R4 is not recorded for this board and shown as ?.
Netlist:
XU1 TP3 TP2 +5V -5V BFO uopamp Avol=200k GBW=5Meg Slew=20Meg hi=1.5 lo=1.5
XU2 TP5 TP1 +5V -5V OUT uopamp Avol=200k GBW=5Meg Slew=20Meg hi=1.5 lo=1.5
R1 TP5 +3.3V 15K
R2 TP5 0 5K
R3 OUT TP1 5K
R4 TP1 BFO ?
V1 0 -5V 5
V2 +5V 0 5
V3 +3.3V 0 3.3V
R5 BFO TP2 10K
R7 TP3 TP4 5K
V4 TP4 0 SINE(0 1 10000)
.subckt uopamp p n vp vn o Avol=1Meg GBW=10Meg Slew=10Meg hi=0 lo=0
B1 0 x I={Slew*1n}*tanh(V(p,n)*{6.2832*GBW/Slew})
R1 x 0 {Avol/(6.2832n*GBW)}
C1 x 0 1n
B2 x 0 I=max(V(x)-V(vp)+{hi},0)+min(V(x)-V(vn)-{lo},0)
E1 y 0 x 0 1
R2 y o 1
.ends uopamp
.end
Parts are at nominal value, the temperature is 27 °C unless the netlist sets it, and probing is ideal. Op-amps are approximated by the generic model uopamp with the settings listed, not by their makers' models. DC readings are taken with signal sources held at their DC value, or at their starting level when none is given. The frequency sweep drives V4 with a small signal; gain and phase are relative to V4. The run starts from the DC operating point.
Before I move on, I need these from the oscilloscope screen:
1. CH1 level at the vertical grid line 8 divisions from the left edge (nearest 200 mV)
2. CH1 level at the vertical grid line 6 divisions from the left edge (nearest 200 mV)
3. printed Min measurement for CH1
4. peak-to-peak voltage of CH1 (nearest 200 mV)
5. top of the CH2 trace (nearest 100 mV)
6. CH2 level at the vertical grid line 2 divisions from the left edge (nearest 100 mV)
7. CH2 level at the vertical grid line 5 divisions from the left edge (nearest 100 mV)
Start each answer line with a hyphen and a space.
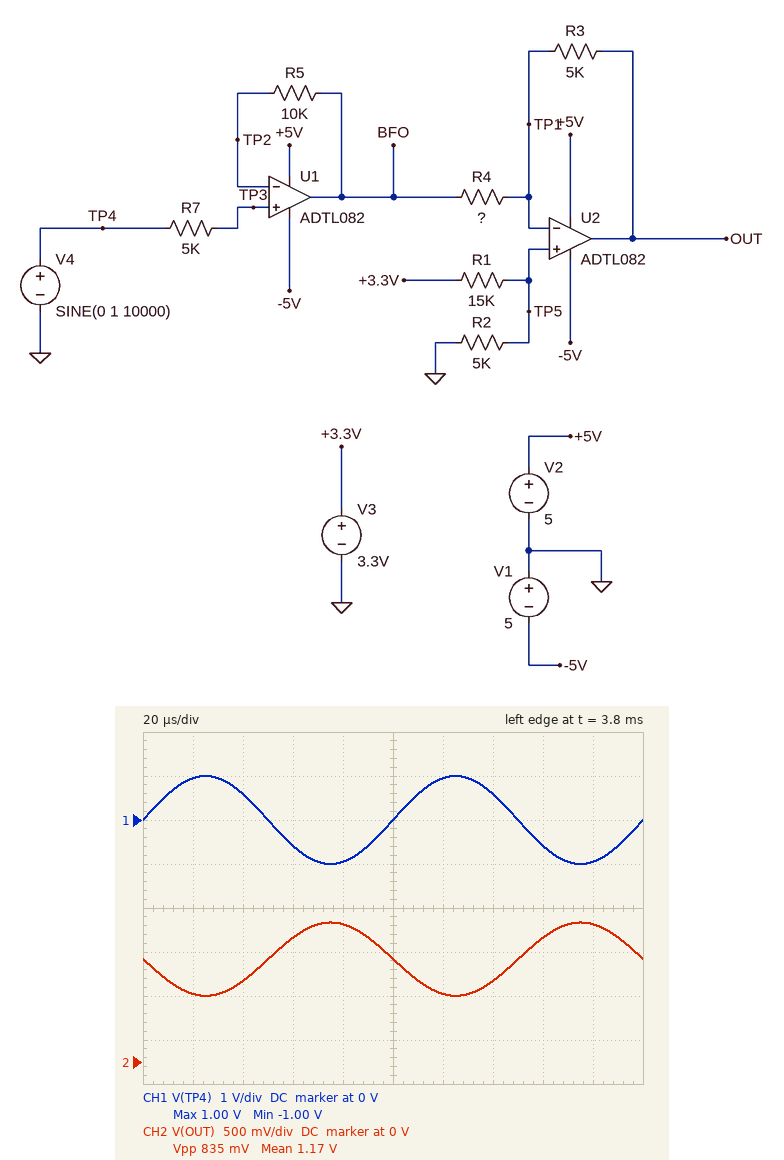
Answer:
- -600 mV
- 1.0 V
- -1.00 V
- 2.0 V
- 1.6 V
- 900 mV
- 1.2 V
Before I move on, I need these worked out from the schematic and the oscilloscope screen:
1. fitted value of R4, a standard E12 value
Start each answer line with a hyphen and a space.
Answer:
- 12 kΩ
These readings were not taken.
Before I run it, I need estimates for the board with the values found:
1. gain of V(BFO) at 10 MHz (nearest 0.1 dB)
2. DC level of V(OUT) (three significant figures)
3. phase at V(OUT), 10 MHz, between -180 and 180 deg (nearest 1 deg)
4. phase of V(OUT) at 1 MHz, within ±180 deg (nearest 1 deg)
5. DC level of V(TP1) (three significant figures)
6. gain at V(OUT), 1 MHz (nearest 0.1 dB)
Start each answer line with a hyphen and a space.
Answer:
- -7.0 dB
- 1.17 V
- 46 deg
- 153 deg
- 825 mV
- -8.1 dB
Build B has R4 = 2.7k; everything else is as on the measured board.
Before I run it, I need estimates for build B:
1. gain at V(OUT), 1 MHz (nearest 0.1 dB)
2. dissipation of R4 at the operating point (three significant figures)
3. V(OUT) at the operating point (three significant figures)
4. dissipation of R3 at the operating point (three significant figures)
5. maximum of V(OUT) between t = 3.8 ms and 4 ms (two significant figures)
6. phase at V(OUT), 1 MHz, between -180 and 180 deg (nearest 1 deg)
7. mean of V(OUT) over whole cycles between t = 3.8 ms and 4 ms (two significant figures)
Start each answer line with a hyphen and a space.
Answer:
- 4.0 dB
- 252 µW
- 2.35 V
- 467 µW
- 3.5 V
- 139 deg
- 2.2 V
